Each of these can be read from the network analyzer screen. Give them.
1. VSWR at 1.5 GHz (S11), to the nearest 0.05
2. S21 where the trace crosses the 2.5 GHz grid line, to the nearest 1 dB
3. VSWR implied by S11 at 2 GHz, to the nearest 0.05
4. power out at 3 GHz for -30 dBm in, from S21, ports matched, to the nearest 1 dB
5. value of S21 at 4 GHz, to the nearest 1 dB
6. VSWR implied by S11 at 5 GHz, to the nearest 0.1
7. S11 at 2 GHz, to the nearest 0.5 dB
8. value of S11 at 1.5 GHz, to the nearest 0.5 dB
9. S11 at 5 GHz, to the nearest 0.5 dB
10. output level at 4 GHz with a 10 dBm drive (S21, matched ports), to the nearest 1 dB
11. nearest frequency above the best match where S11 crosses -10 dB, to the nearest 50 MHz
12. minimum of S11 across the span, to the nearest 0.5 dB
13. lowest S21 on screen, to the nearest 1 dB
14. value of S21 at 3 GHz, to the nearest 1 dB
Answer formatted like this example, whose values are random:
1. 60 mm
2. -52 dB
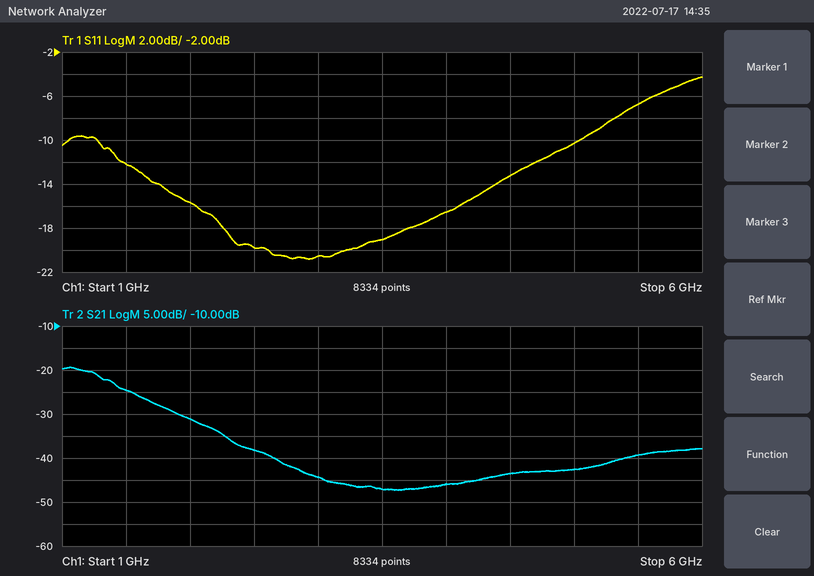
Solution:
1. 1.65
2. -38 dB
3. 1.40
4. -74 dBm
5. -46 dB
6. 1.9
7. -15.5 dB
8. -12.0 dB
9. -10.5 dB
10. -36 dBm
11. 5.05 GHz
12. -21.0 dB
13. -47 dB
14. -44 dB
